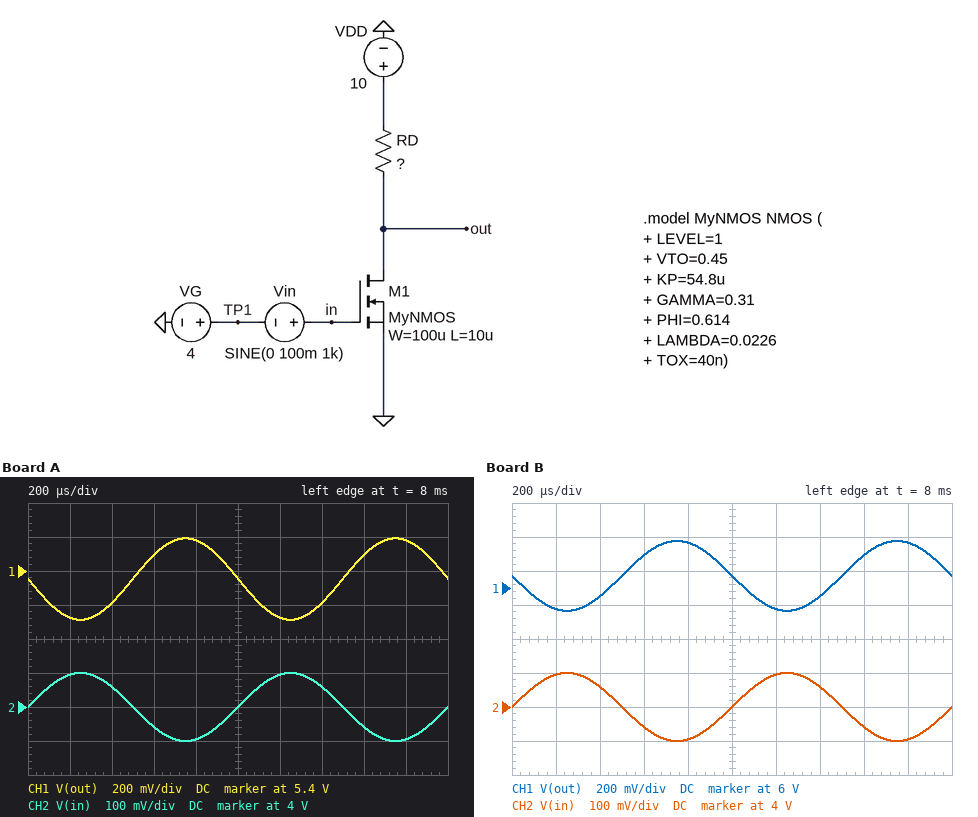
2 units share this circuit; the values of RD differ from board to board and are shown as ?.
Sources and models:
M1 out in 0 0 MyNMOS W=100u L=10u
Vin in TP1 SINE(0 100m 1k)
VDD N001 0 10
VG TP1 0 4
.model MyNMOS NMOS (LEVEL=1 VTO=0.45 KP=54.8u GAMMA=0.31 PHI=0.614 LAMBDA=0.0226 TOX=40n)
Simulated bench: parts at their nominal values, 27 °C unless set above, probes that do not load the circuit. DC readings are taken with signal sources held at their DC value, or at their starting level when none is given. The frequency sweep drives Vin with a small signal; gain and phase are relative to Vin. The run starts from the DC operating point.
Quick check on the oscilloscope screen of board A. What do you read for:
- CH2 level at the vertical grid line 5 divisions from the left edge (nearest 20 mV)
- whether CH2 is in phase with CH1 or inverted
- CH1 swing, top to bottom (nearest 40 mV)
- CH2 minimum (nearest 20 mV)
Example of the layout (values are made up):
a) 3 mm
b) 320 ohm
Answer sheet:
a) 4.00 V
b) inverted
c) 480 mV
d) 3.90 V
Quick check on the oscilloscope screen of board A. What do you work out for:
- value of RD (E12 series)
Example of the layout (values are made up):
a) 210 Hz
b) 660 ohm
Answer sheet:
a) 1.2 kΩ
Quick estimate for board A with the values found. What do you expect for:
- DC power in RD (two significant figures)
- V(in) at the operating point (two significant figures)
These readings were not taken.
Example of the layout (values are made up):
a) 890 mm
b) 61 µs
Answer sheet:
a) 18 mW
b) 4.0 V
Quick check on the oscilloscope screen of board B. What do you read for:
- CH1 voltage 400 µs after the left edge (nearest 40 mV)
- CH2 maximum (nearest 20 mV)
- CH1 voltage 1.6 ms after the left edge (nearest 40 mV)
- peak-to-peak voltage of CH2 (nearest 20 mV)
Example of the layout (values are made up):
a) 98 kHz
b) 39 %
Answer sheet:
a) 5.96 V
b) 4.10 V
c) 6.20 V
d) 200 mV
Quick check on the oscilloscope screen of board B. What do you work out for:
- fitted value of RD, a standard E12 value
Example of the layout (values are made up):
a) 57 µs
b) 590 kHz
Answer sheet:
a) 1 kΩ
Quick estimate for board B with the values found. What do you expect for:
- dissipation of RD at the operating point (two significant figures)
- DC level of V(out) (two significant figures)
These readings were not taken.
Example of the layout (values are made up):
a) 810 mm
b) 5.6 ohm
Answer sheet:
a) 15 mW
b) 6.1 V
